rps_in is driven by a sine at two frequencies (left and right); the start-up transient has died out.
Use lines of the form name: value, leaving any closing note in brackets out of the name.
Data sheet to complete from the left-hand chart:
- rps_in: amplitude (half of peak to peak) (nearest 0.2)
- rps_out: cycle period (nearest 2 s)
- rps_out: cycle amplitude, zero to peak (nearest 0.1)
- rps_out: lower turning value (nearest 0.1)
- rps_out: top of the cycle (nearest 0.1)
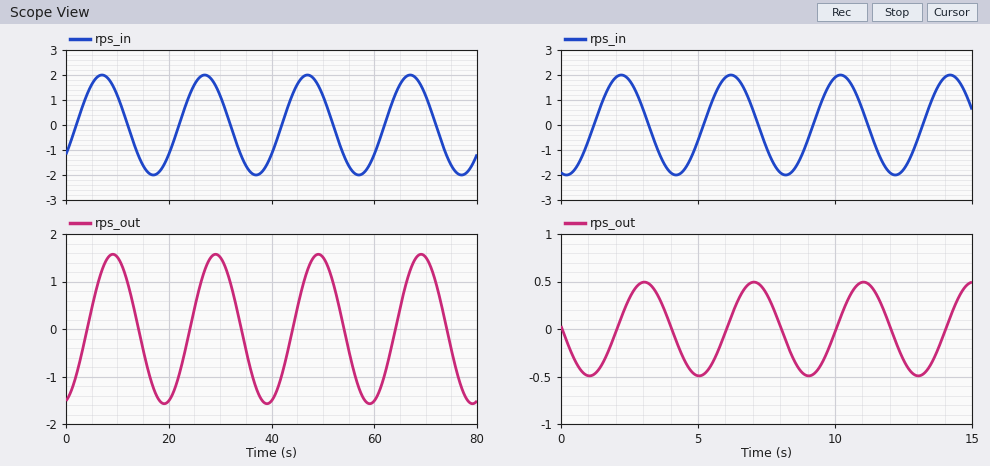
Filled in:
rps_in: amplitude (half of peak to peak): 2.0
rps_out: cycle period: 20 s
rps_out: cycle amplitude, zero to peak: 1.6
rps_out: lower turning value: -1.6
rps_out: top of the cycle: 1.6
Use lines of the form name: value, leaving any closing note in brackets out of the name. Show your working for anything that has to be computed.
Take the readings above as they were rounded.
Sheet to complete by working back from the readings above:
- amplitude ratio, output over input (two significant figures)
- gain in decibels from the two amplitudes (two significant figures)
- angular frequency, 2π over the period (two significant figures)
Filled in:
amplitude ratio, output over input: 1.6 / 2 = 0.80
gain in decibels from the two amplitudes: 20 log10(1.6 / 2) = -1.9 dB
angular frequency, 2π over the period: 2π / 20 = 0.31 rad/s
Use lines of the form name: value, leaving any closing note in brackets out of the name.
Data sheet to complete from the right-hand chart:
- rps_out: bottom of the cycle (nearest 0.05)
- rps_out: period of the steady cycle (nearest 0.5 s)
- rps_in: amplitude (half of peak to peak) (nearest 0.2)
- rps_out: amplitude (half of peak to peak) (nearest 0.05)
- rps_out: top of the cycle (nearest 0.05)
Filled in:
rps_out: bottom of the cycle: -0.50
rps_out: period of the steady cycle: 4.0 s
rps_in: amplitude (half of peak to peak): 2.0
rps_out: amplitude (half of peak to peak): 0.50
rps_out: top of the cycle: 0.50
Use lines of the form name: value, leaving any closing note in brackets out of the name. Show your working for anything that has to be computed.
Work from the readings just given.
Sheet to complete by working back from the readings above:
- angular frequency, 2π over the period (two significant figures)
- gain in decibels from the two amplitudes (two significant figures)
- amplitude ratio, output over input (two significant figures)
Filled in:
angular frequency, 2π over the period: 2π / 4 = 1.6 rad/s
gain in decibels from the two amplitudes: 20 log10(0.5 / 2) = -12 dB
amplitude ratio, output over input: 0.5 / 2 = 0.25
